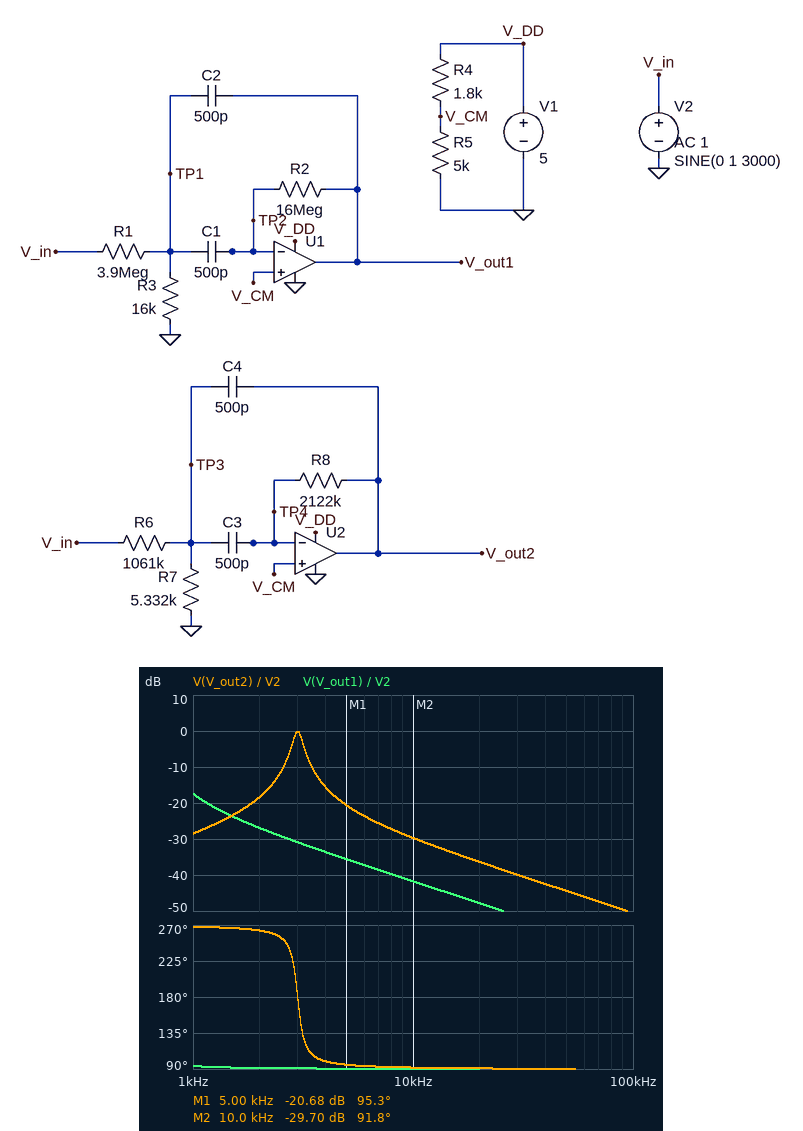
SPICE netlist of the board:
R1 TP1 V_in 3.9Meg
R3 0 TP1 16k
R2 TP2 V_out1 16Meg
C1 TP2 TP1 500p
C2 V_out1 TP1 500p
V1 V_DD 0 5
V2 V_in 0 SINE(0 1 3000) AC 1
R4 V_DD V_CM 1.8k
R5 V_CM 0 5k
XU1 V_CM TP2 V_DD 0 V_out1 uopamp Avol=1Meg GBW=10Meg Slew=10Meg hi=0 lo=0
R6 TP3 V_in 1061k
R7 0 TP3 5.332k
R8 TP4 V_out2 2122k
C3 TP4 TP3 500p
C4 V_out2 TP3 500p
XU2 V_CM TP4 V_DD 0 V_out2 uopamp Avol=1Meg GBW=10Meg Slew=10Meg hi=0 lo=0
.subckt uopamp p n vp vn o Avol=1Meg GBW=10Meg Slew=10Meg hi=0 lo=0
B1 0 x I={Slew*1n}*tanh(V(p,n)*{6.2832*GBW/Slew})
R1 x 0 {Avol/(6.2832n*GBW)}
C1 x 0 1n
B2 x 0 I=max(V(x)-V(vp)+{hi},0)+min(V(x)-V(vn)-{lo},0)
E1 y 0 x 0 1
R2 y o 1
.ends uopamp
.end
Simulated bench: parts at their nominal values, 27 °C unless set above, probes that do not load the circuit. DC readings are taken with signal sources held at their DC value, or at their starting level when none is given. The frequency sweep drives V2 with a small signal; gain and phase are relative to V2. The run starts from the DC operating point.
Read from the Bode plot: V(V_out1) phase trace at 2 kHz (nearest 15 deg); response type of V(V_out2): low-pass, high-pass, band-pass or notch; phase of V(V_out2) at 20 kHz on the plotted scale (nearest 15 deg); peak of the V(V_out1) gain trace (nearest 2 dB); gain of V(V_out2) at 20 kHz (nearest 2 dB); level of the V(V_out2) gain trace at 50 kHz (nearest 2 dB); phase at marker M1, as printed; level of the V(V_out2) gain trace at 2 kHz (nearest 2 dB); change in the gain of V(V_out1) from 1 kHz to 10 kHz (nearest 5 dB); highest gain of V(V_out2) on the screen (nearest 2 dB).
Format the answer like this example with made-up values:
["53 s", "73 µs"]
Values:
["90 deg", "band-pass", "90 deg", "-18 dB", "-36 dB", "-44 dB", "95.3 deg", "-18 dB", "-25 dB", "0 dB"]
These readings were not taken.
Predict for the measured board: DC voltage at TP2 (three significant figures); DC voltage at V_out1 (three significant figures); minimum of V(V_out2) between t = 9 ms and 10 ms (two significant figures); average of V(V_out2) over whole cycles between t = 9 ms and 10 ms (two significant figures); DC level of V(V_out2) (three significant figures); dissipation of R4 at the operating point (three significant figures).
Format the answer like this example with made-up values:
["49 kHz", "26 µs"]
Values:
["3.68 V", "3.68 V", "2.7 V", "3.7 V", "3.68 V", "973 µW"]
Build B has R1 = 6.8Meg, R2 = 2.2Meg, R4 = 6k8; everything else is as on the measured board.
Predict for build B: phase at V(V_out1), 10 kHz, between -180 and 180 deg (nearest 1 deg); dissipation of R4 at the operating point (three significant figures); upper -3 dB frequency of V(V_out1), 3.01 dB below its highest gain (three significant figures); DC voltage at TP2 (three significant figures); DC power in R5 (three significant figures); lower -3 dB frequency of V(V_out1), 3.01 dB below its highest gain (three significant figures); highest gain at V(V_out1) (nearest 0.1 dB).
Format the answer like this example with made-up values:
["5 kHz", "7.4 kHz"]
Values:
["92 deg", "1.22 mW", "1.85 kHz", "2.12 V", "898 µW", "1.56 kHz", "-15.8 dB"]
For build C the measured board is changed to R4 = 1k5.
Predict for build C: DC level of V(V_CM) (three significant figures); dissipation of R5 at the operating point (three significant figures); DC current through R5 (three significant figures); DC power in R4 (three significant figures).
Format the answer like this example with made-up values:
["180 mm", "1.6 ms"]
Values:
["3.85 V", "2.96 mW", "769 µA", "888 µW"]
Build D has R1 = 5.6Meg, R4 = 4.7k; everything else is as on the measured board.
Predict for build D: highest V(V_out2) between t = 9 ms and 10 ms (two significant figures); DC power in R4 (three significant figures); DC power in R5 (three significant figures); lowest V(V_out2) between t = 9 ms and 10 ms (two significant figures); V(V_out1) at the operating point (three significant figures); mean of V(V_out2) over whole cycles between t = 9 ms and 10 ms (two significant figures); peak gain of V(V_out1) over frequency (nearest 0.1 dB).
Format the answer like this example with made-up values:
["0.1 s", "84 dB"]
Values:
["3.6 V", "1.25 mW", "1.33 mW", "1.6 V", "2.58 V", "2.6 V", "3.1 dB"]
